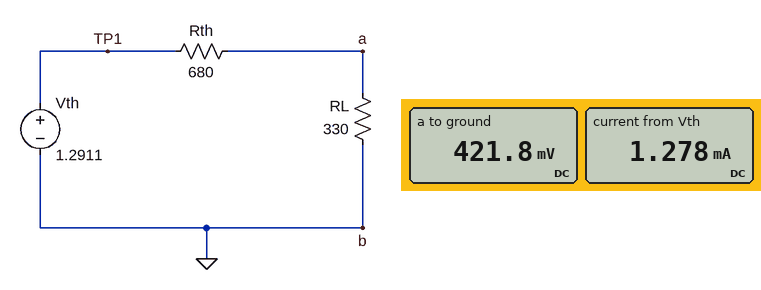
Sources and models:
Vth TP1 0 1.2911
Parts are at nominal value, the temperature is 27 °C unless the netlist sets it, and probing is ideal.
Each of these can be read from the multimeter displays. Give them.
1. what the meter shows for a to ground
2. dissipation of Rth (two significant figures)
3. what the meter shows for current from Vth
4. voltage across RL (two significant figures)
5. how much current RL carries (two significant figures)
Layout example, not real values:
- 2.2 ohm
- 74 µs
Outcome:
- 421.8 mV
- 1.1 mW
- 1.278 mA
- 420 mV
- 1.3 mA
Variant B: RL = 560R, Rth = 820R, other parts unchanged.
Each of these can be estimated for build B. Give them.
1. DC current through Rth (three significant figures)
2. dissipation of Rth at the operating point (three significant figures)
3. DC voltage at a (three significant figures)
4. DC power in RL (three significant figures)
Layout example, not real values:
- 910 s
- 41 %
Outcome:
- 936 µA
- 718 µW
- 524 mV
- 490 µW
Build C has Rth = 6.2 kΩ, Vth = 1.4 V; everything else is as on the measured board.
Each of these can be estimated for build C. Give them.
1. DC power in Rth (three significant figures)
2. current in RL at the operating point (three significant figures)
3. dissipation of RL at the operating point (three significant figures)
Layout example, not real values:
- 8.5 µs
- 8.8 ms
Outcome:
- 285 µW
- 214 µA
- 15.2 µW
